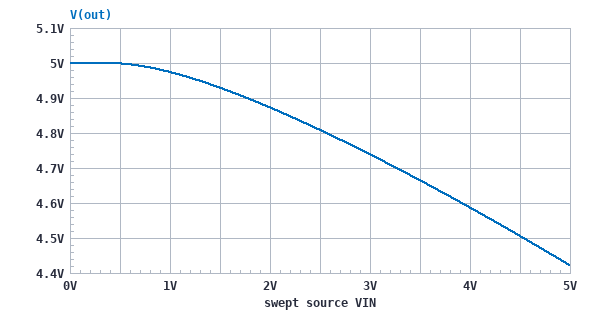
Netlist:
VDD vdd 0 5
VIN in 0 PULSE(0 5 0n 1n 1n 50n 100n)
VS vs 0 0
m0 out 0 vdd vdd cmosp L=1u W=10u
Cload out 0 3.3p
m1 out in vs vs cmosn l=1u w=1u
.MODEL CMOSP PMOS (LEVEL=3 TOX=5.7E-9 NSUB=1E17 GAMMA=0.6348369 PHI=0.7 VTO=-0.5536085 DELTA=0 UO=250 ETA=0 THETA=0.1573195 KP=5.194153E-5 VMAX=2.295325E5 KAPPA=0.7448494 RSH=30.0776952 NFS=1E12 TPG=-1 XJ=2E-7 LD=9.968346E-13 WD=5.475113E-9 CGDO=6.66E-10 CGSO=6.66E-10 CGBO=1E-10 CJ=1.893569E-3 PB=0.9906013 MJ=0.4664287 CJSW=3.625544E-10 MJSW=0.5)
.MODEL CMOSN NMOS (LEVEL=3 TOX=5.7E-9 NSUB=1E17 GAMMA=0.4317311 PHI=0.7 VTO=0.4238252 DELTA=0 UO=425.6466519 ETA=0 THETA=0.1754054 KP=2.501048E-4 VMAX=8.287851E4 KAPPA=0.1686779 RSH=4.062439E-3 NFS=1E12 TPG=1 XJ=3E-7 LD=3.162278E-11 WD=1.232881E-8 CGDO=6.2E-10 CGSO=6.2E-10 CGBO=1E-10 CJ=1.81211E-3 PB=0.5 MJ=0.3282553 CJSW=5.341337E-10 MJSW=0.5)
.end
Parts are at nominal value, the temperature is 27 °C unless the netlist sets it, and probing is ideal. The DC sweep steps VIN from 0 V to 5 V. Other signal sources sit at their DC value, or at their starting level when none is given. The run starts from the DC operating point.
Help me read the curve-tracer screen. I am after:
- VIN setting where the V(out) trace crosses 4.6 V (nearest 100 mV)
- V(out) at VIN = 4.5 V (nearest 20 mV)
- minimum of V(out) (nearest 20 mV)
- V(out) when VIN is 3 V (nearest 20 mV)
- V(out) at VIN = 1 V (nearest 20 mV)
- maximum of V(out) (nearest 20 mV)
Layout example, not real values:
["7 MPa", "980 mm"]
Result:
["3.9 V", "4.50 V", "4.42 V", "4.74 V", "4.98 V", "5.00 V"]
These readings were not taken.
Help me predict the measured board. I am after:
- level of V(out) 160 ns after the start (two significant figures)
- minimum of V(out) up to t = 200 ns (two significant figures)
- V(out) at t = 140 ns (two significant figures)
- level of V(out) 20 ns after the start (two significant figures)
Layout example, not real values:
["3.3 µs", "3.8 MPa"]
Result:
["5.0 V", "4.4 V", "4.4 V", "4.4 V"]
